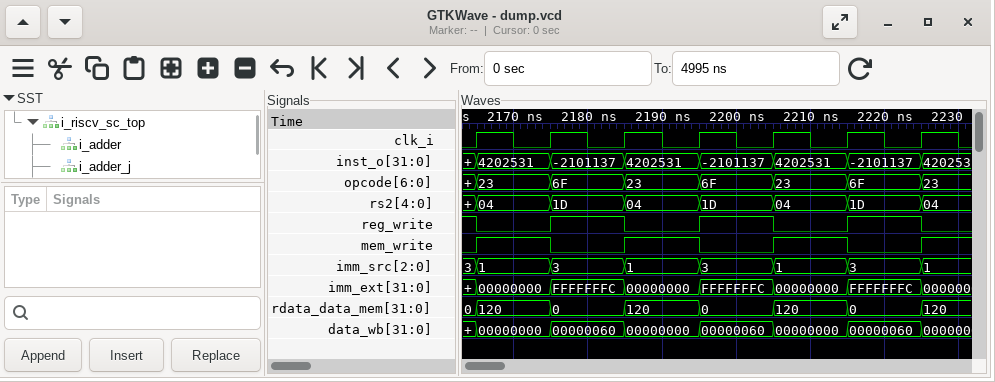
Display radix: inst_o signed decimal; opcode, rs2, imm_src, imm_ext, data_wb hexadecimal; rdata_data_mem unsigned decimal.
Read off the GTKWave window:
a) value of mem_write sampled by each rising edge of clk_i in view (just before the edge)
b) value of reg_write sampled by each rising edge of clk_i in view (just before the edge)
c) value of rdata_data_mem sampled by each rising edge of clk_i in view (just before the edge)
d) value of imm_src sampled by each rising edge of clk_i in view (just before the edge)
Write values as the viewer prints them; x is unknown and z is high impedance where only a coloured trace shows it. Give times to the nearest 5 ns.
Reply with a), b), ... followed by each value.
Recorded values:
a) 0 1 0 1 0 1 0
b) 1 0 1 0 1 0 1
c) 0, 120, 0, 120, 0, 120, 0
d) 3, 1, 3, 1, 3, 1, 3
